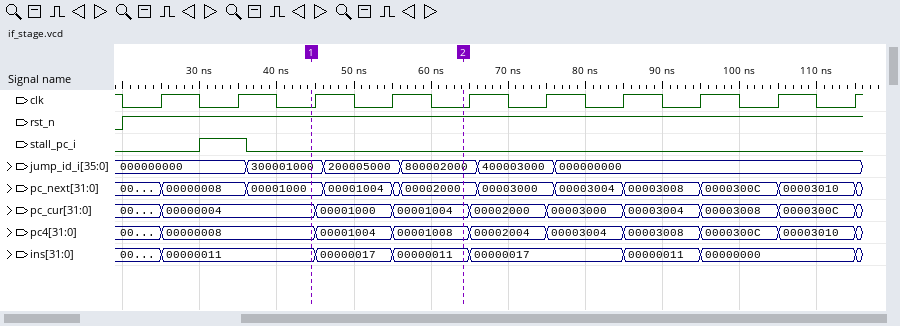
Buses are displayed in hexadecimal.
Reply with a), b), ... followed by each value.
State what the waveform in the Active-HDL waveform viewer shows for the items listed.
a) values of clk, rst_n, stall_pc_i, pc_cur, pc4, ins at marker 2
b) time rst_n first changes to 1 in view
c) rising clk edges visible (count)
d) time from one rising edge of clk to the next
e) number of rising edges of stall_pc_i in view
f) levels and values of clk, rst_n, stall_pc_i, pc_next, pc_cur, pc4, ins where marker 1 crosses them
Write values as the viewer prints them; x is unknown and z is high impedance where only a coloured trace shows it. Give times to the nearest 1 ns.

a) clk=0, rst_n=1, stall_pc_i=0, pc_cur=00001004, pc4=00001008, ins=00000011
b) 20 ns
c) 10
d) 10 ns
e) 1
f) clk=0, rst_n=1, stall_pc_i=0, pc_next=00001000, pc_cur=00000004, pc4=00000008, ins=00000011
